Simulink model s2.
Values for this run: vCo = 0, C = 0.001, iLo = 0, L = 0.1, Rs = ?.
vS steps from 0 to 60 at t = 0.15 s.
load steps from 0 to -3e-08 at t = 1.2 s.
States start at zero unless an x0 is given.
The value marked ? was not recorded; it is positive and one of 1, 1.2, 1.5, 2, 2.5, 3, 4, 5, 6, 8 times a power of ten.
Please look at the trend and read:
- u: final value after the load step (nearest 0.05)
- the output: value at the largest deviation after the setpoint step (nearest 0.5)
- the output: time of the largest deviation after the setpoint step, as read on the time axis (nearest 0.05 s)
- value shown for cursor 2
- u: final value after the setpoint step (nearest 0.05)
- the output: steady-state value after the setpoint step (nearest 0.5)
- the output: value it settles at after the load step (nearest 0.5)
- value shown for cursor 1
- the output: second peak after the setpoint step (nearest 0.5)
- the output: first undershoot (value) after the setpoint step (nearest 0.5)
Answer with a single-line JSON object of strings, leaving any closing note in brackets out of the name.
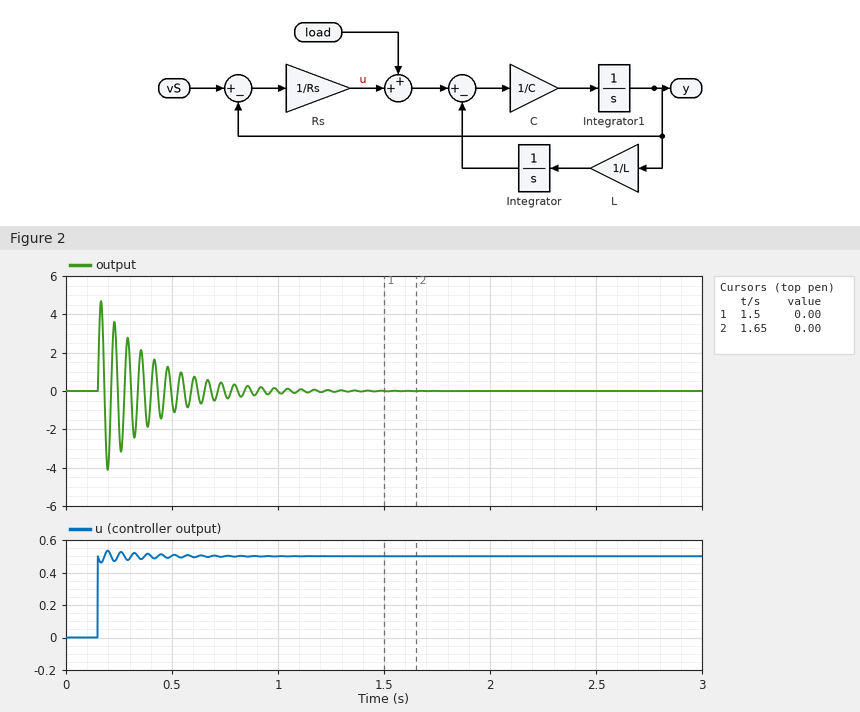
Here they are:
{"u: final value after the load step": "0.50", "the output: value at the largest deviation after the setpoint step": "4.5", "the output: time of the largest deviation after the setpoint step, as read on the time axis": "0.15 s", "value shown for cursor 2": "0.00", "u: final value after the setpoint step": "0.50", "the output: steady-state value after the setpoint step": "0.0", "the output: value it settles at after the load step": "0.0", "value shown for cursor 1": "0.00", "the output: second peak after the setpoint step": "3.5", "the output: first undershoot (value) after the setpoint step": "-4.0"}
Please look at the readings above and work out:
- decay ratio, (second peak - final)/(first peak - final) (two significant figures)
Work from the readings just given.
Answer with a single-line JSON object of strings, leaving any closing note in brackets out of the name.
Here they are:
{"decay ratio, (second peak - final)/(first peak - final)": "0.78"}
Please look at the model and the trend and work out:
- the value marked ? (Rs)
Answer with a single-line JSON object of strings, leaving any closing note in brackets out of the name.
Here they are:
{"the value marked ?": "120"}
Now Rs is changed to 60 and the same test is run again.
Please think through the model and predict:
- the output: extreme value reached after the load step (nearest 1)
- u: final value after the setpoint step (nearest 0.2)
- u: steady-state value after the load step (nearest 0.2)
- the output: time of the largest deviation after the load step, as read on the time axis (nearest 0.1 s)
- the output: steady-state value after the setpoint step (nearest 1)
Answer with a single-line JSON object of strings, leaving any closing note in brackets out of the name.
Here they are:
{"the output: extreme value reached after the load step": "0", "u: final value after the setpoint step": "1.0", "u: steady-state value after the load step": "1.0", "the output: time of the largest deviation after the load step, as read on the time axis": "1.2 s", "the output: steady-state value after the setpoint step": "0"}
